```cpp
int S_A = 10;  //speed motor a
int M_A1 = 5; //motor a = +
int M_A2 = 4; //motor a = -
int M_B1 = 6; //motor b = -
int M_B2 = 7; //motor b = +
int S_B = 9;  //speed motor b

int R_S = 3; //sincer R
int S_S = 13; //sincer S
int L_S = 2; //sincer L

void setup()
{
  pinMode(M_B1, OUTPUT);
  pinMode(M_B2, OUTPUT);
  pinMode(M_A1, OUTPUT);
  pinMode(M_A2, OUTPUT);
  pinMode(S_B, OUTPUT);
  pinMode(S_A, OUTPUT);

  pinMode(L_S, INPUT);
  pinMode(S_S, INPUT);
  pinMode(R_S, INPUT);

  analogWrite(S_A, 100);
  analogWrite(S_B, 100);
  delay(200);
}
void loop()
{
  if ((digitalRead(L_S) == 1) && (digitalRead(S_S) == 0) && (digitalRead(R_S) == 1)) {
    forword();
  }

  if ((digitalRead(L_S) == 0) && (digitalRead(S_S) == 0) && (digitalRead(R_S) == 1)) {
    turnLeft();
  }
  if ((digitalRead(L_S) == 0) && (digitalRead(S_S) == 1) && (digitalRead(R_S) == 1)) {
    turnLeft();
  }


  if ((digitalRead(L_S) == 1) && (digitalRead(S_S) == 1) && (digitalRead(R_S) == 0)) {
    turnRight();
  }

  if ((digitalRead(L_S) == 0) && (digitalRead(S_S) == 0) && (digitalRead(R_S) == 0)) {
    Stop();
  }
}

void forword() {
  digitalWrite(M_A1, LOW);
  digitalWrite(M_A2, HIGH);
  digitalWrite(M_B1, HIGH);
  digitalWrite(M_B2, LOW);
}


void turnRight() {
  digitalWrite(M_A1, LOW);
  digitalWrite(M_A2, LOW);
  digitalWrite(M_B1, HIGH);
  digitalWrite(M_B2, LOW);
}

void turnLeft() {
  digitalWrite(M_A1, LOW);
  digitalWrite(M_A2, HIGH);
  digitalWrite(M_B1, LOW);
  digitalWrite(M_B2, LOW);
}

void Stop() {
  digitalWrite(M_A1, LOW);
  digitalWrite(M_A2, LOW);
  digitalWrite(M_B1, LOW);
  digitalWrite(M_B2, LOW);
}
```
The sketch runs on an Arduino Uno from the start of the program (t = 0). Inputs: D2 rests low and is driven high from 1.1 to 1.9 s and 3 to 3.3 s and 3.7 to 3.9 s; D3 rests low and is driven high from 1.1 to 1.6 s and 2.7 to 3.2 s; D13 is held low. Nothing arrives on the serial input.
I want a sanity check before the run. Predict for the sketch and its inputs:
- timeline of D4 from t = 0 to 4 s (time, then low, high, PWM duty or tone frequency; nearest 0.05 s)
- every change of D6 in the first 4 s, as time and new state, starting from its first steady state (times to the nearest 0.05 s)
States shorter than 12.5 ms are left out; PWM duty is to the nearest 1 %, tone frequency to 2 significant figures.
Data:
0 s low; 1.1 s high; 1.9 s low; 2.7 s high; 3.3 s low
0 s low; 1.1 s high; 1.9 s low; 3 s high; 3.3 s low
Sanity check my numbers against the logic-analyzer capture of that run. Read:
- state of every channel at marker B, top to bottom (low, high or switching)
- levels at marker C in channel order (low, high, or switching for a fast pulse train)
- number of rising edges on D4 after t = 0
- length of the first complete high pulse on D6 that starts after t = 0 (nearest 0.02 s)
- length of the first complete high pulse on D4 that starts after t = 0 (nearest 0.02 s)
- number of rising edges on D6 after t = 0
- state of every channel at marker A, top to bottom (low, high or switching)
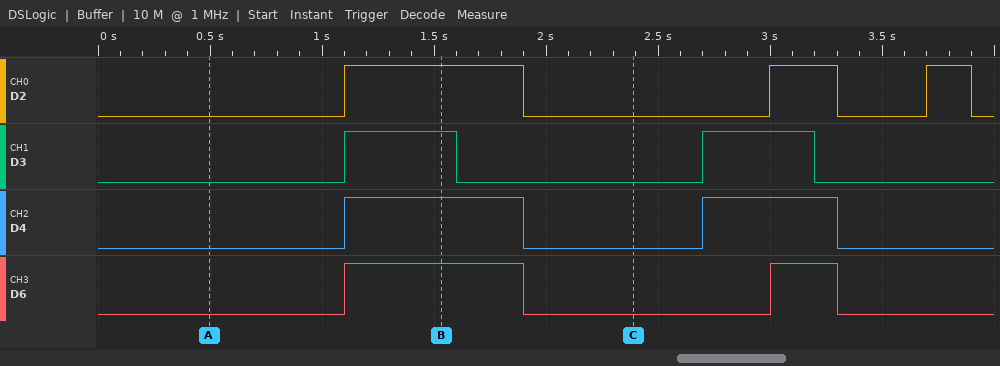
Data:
D2 high, D3 high, D4 high, D6 high
D2 low, D3 low, D4 low, D6 low
2
0.80 s
0.80 s
2
D2 low, D3 low, D4 low, D6 low
